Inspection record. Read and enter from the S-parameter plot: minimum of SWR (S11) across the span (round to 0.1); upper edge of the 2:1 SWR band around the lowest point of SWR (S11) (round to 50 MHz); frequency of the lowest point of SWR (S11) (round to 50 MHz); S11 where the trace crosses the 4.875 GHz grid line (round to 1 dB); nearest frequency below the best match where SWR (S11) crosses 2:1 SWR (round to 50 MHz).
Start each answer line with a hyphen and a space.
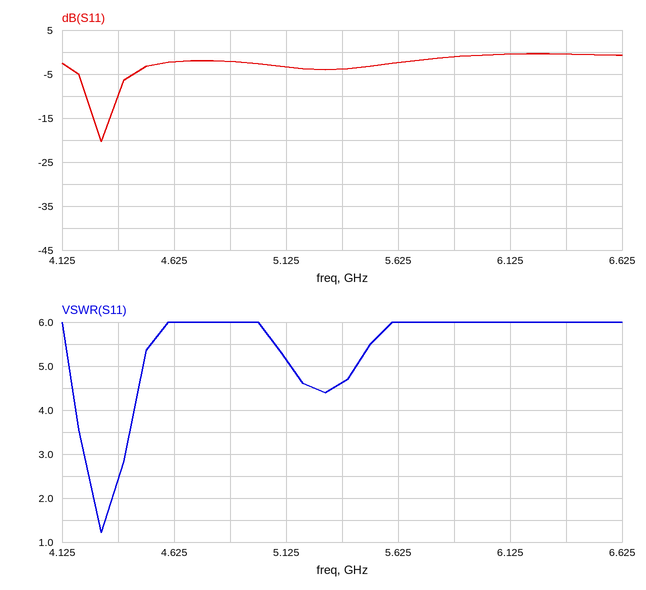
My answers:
- 1.2
- 4.35 GHz
- 4.30 GHz
- -2 dB
- 4.25 GHz
